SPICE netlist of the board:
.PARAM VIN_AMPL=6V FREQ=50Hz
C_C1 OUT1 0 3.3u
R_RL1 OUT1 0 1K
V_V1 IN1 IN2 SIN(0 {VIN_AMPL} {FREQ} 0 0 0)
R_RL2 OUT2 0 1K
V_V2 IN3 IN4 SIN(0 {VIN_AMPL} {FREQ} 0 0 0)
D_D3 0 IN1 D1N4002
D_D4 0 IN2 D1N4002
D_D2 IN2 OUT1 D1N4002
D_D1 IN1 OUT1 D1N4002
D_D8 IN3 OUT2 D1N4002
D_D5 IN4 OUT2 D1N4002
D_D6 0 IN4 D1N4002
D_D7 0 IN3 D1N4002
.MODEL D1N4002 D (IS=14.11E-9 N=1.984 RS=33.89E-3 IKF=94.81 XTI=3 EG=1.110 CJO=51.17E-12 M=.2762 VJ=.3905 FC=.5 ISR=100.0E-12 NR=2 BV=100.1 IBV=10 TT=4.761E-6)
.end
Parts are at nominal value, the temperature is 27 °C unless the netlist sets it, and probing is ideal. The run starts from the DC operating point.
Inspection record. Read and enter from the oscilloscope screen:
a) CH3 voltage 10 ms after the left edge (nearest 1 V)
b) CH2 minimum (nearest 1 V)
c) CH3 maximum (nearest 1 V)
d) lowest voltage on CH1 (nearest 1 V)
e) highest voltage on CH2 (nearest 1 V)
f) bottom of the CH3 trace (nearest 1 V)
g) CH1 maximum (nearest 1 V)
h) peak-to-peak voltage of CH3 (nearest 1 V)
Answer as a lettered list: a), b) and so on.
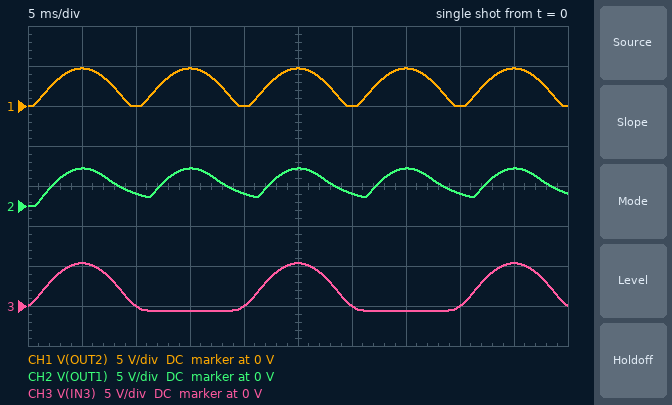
a) 0 V
b) 0 V
c) 5 V
d) 0 V
e) 5 V
f) -1 V
g) 5 V
h) 6 V
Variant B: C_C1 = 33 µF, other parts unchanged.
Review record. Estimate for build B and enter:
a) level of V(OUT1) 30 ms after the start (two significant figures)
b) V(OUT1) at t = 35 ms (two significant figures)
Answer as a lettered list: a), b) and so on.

a) 4.1 V
b) 4.6 V
